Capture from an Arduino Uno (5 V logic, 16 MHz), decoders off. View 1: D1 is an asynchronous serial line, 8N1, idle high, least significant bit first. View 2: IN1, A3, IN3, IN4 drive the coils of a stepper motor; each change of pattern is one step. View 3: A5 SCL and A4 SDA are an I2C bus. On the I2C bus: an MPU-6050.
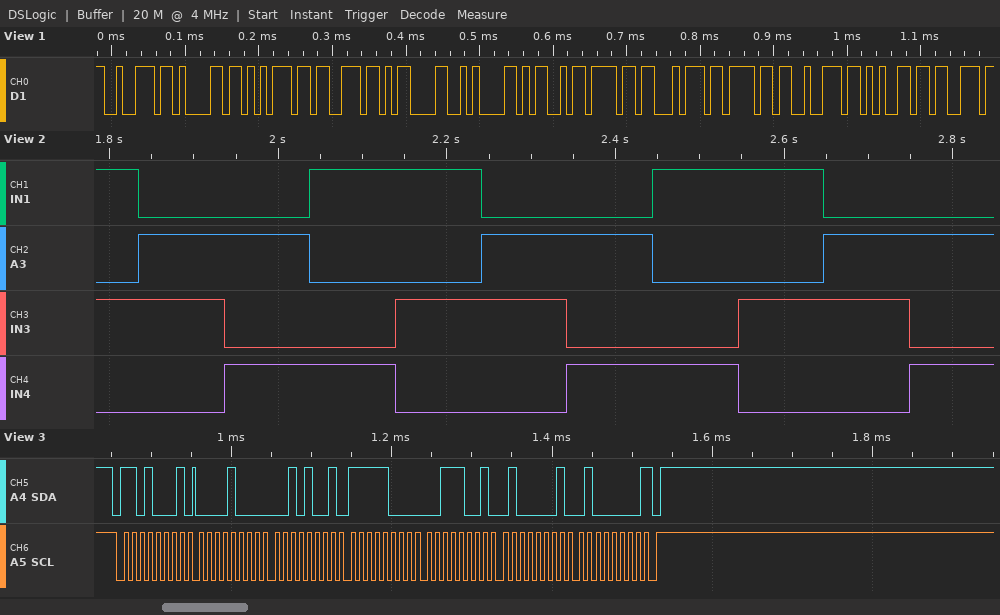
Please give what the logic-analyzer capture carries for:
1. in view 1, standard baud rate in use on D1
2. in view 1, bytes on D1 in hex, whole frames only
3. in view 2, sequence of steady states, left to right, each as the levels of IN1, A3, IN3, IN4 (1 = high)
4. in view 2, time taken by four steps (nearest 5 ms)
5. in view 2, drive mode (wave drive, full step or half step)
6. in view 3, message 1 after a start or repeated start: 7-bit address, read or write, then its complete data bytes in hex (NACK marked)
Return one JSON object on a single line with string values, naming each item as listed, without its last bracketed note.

{"in view 1, standard baud rate in use on D1": "115200 baud", "in view 1, bytes on D1 in hex, whole frames only": "0x72 0x61 0x75 0x73 0x0D 0x0A 0x4D 0x6F 0x74 0x6F 0x72 0x65 0x73", "in view 2, sequence of steady states, left to right, each as the levels of IN1, A3, IN3, IN4": "1010 0110 0101 1001 1010 0110 0101 1001 1010 0110 0101", "in view 2, time taken by four steps": "405 ms", "in view 2, drive mode": "full step", "in view 3, message 1 after a start or repeated start: 7-bit address, read or write, then its complete data bytes in hex": "0x68 read: 08 29 F8 39 41 40 NACK"}
